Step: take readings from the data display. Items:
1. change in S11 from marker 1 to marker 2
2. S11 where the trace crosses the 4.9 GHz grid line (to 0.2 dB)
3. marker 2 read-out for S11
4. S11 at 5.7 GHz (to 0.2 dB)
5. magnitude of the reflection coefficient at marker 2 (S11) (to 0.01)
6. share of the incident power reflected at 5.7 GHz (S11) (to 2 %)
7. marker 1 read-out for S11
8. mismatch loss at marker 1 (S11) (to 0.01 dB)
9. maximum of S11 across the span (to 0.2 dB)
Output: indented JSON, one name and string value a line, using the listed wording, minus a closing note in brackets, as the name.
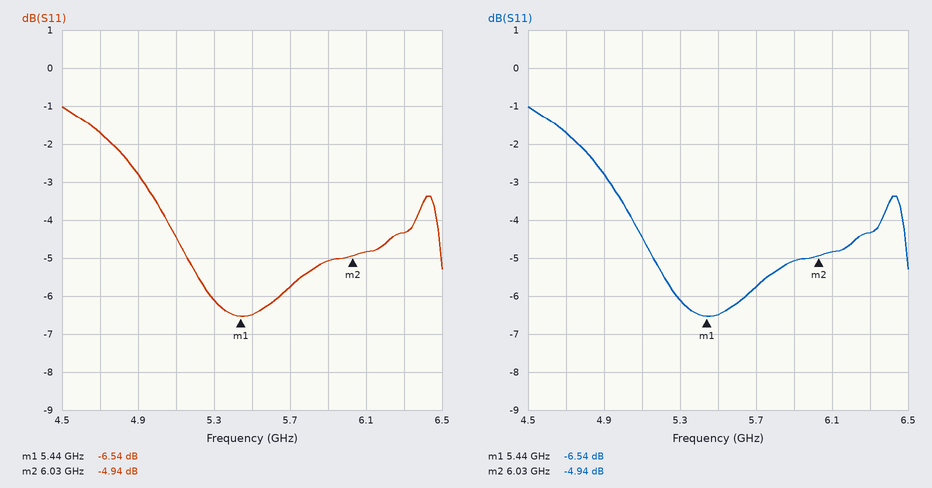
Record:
{
  "change in S11 from marker 1 to marker 2": "1.60 dB",
  "S11 where the trace crosses the 4.9 GHz grid line": "-2.8 dB",
  "marker 2 read-out for S11": "-4.94 dB",
  "S11 at 5.7 GHz": "-5.8 dB",
  "magnitude of the reflection coefficient at marker 2 (S11)": "0.57",
  "share of the incident power reflected at 5.7 GHz (S11)": "26 %",
  "marker 1 read-out for S11": "-6.54 dB",
  "mismatch loss at marker 1 (S11)": "1.09 dB",
  "maximum of S11 across the span": "-1.0 dB"
}
